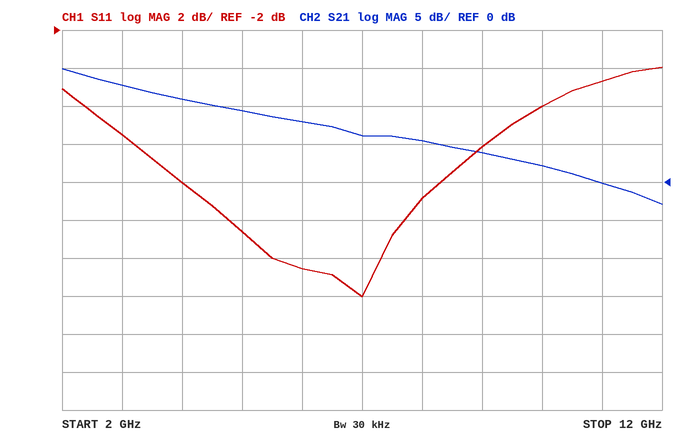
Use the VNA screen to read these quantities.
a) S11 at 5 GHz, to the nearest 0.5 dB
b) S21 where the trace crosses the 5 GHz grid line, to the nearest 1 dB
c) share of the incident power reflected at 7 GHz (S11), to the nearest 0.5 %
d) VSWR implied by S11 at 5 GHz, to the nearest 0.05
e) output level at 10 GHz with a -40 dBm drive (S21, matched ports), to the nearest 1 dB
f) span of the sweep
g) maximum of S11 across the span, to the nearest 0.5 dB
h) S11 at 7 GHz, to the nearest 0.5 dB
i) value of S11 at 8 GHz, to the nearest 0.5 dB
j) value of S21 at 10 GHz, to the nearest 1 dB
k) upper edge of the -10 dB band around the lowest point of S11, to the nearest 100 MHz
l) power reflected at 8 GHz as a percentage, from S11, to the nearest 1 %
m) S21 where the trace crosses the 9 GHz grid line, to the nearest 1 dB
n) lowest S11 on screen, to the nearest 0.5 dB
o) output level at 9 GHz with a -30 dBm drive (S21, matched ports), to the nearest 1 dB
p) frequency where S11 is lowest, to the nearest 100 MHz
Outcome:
-12.5 dB
9 dB
2.5 %
1.60
-38 dBm
10 GHz
-4.0 dB
-16.0 dB
-11.0 dB
2 dB
8.3 GHz
8 %
4 dB
-16.0 dB
-26 dBm
7.0 GHz
